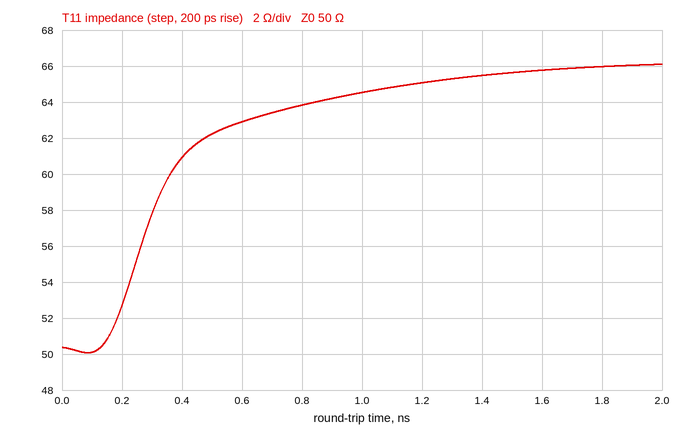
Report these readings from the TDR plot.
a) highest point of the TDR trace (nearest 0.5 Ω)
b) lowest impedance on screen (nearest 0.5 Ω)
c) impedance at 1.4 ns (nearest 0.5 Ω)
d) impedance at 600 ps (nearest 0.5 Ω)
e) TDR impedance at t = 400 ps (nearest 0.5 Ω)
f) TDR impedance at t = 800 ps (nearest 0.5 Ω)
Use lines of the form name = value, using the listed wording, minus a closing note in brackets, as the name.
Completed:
highest point of the TDR trace = 66.0 Ω
lowest impedance on screen = 50.0 Ω
impedance at 1.4 ns = 65.5 Ω
impedance at 600 ps = 63.0 Ω
TDR impedance at t = 400 ps = 61.0 Ω
TDR impedance at t = 800 ps = 64.0 Ω
